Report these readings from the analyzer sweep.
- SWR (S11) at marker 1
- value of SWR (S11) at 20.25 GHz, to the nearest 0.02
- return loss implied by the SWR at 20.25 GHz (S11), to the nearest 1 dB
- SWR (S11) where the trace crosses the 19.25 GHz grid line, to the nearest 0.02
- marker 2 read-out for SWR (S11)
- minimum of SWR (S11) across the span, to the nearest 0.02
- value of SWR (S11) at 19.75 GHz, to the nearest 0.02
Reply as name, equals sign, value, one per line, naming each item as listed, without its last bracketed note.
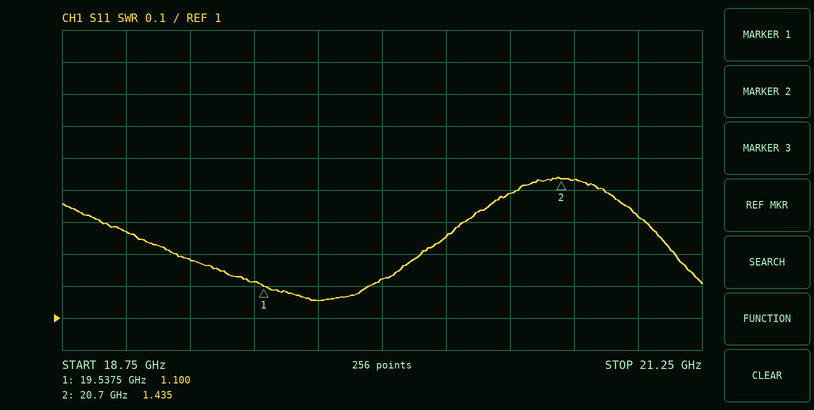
SWR (S11) at marker 1 = 1.100
value of SWR (S11) at 20.25 GHz, to the nearest 0.02 = 1.26
return loss implied by the SWR at 20.25 GHz (S11), to the nearest 1 dB = 19 dB
SWR (S11) where the trace crosses the 19.25 GHz grid line, to the nearest 0.02 = 1.18
marker 2 read-out for SWR = 1.435
minimum of SWR (S11) across the span, to the nearest 0.02 = 1.06
value of SWR (S11) at 19.75 GHz, to the nearest 0.02 = 1.06
